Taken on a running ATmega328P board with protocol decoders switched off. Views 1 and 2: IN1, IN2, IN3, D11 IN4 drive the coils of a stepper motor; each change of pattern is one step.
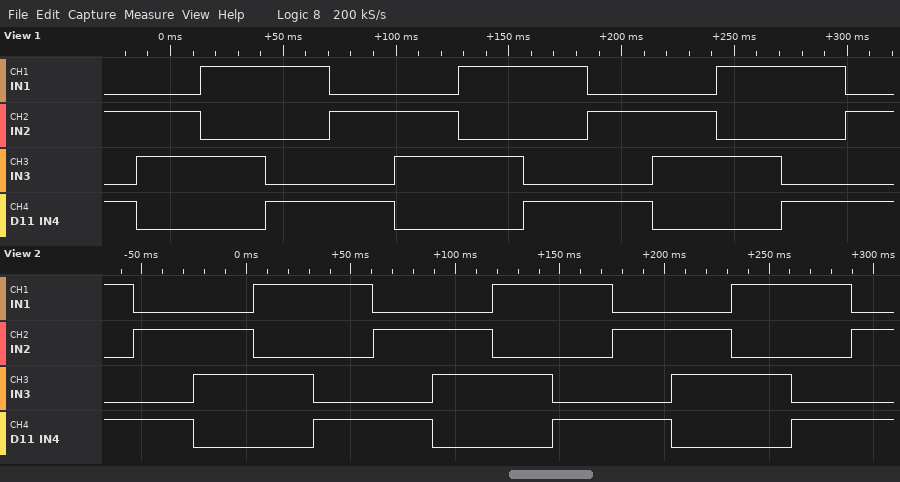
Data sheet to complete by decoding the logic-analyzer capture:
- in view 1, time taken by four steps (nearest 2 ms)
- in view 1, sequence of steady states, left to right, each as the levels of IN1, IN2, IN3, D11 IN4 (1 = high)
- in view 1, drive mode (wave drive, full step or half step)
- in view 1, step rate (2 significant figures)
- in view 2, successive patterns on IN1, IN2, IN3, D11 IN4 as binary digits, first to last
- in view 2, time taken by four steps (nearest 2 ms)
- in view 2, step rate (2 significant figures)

114 ms
0101 0110 1010 1001 0101 0110 1010 1001 0101 0110 1010 1001 0101
full step
35 steps/s
1001 0101 0110 1010 1001 0101 0110 1010 1001 0101 0110 1010 1001 0101
114 ms
35 steps/s
